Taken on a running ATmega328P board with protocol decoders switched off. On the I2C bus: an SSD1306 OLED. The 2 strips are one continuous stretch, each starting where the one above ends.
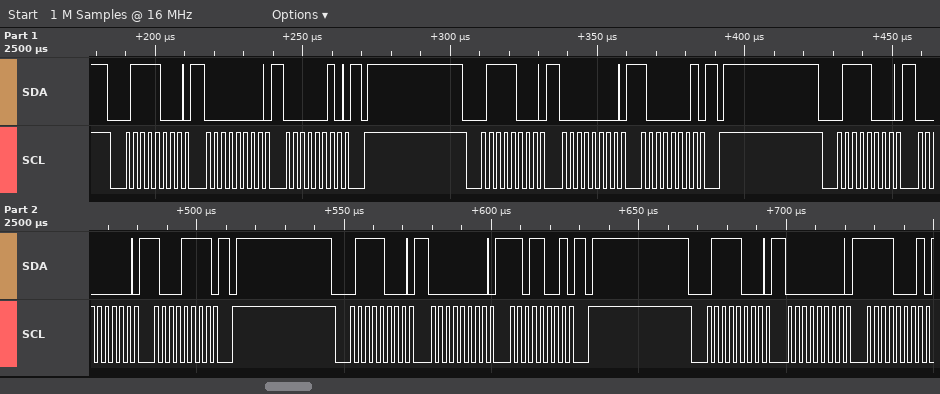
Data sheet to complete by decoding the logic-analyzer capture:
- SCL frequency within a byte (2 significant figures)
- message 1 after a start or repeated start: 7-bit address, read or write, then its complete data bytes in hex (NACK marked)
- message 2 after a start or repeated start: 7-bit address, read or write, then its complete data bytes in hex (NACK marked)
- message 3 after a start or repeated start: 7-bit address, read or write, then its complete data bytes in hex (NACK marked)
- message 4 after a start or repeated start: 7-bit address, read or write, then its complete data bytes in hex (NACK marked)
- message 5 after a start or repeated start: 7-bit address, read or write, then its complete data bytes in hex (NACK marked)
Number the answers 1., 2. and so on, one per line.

1. 400 kHz
2. 0x3C write: 00 02
3. 0x3C write: 00 81
4. 0x3C write: 00 8F
5. 0x3C write: 00 D9
6. 0x3C write: 00 F1
